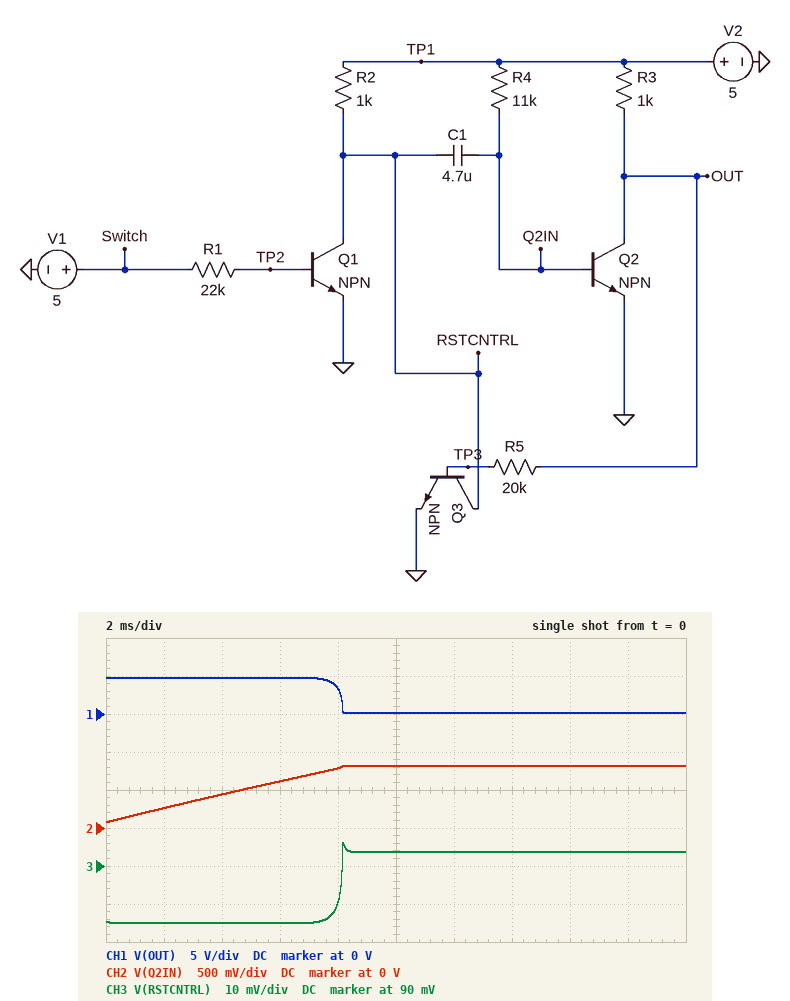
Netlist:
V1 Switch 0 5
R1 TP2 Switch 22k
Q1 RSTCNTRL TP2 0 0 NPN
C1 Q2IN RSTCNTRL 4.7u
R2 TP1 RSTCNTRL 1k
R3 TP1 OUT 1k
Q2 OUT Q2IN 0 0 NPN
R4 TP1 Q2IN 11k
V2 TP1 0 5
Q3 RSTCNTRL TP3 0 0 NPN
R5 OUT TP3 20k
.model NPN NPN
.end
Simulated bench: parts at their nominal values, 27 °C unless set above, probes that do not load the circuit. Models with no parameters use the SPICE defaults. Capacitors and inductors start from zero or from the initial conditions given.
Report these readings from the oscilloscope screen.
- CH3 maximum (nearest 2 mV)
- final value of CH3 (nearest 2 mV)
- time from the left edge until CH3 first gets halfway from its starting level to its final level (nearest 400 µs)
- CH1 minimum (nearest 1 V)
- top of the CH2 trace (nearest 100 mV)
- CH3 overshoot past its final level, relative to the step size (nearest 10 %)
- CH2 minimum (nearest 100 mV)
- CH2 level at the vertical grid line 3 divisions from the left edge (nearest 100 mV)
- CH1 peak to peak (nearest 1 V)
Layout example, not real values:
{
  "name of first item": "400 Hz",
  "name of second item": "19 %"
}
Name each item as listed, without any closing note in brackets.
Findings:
{
  "CH3 maximum": "96 mV",
  "final value of CH3": "94 mV",
  "time from the left edge until CH3 first gets halfway from its starting level to its final level": "8.0 ms",
  "CH1 minimum": "0 V",
  "top of the CH2 trace": "800 mV",
  "CH3 overshoot past its final level, relative to the step size": "10 %",
  "CH2 minimum": "100 mV",
  "CH2 level at the vertical grid line 3 divisions from the left edge": "600 mV",
  "CH1 peak to peak": "5 V"
}
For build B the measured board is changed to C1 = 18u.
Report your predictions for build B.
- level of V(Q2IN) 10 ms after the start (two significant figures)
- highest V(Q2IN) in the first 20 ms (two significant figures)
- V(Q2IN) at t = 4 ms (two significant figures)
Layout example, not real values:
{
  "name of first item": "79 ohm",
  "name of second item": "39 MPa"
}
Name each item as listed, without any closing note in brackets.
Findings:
{
  "level of V(Q2IN) 10 ms after the start": "320 mV",
  "highest V(Q2IN) in the first 20 ms": "550 mV",
  "V(Q2IN) at t = 4 ms": "170 mV"
}
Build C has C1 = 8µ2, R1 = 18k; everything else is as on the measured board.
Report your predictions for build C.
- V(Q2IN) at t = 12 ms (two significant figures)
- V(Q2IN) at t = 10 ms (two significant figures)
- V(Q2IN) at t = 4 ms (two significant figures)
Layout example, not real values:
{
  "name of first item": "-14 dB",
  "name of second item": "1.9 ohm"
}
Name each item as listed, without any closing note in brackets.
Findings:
{
  "V(Q2IN) at t = 12 ms": "690 mV",
  "V(Q2IN) at t = 10 ms": "590 mV",
  "V(Q2IN) at t = 4 ms": "290 mV"
}
